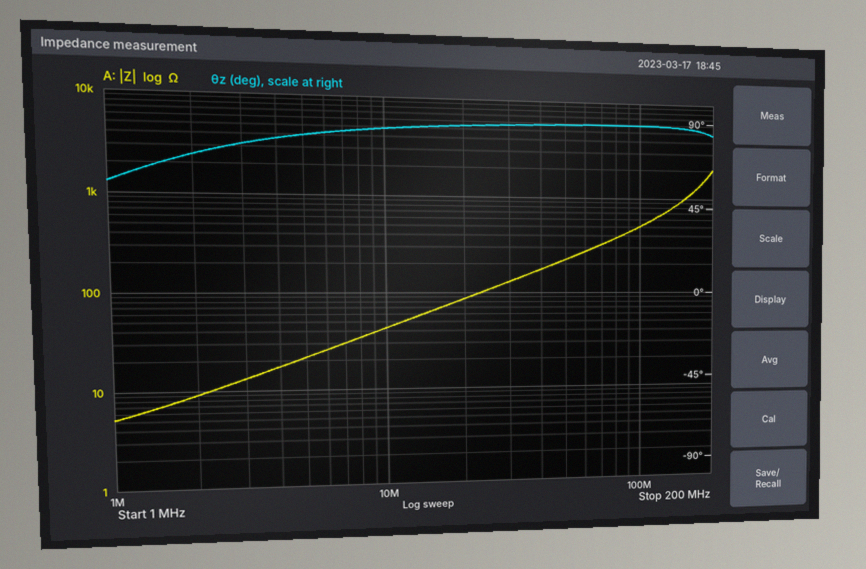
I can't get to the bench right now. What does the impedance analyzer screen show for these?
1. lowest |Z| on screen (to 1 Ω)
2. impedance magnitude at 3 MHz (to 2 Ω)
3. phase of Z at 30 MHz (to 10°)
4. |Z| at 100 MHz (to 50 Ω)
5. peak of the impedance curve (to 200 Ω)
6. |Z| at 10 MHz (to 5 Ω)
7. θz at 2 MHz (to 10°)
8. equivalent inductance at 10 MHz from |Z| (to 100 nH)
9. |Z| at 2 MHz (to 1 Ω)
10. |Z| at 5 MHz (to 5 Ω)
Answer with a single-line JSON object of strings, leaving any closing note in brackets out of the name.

{"lowest |Z| on screen": "5 Ω", "impedance magnitude at 3 MHz": "14 Ω", "phase of Z at 30 MHz": "90°", "|Z| at 100 MHz": "500 Ω", "peak of the impedance curve": "2.0 kΩ", "|Z| at 10 MHz": "45 Ω", "θz at 2 MHz": "70°", "equivalent inductance at 10 MHz from |Z|": "700 nH", "|Z| at 2 MHz": "9 Ω", "|Z| at 5 MHz": "20 Ω"}
